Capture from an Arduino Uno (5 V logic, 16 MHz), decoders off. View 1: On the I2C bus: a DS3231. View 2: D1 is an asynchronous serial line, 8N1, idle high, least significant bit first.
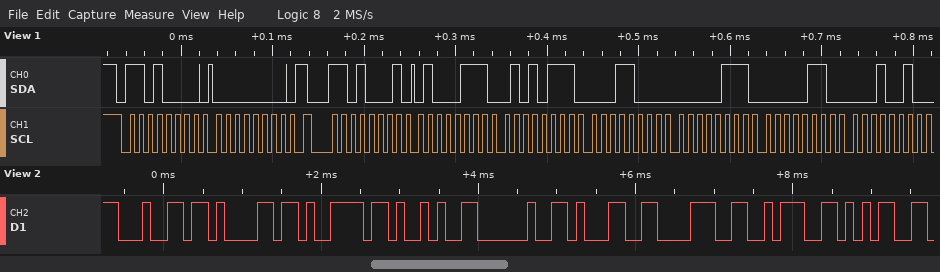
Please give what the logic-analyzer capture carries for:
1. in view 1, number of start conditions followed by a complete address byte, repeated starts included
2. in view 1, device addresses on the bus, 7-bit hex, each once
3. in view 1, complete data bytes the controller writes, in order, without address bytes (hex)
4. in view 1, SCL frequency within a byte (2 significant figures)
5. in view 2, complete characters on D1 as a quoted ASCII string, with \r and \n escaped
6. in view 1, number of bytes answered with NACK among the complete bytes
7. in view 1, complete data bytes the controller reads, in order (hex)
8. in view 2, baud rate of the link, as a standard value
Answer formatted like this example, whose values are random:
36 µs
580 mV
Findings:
2
0x68
00
100 kHz
"day) 18:5"
0
47 57 18 07 06 12
9600 baud
